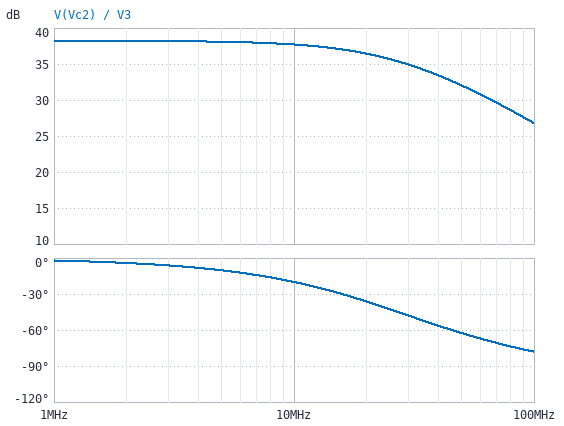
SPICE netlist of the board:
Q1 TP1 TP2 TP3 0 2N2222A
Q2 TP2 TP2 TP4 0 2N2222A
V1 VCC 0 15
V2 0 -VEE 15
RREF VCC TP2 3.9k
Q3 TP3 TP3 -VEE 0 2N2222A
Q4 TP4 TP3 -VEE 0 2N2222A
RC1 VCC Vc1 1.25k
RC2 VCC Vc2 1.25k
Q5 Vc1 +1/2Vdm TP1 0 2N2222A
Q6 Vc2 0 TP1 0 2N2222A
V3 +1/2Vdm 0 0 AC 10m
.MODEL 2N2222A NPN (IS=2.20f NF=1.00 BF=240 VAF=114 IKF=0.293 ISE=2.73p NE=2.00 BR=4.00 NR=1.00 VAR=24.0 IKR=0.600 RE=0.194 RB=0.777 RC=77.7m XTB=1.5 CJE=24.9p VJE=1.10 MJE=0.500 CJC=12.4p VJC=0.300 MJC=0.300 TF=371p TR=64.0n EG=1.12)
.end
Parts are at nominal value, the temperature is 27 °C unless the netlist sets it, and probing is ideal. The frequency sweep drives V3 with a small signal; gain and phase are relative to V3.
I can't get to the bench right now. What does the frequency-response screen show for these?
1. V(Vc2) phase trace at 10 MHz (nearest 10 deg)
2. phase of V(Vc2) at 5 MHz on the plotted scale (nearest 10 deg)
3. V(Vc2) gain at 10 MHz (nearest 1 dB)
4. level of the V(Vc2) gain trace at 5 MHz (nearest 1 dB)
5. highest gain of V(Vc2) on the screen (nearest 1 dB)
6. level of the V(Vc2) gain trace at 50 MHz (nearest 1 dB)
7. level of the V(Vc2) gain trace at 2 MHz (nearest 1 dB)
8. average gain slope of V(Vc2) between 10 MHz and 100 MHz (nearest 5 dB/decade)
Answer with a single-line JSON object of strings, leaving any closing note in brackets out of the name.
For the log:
{"V(Vc2) phase trace at 10 MHz": "-20 deg", "phase of V(Vc2) at 5 MHz on the plotted scale": "-10 deg", "V(Vc2) gain at 10 MHz": "38 dB", "level of the V(Vc2) gain trace at 5 MHz": "38 dB", "highest gain of V(Vc2) on the screen": "38 dB", "level of the V(Vc2) gain trace at 50 MHz": "32 dB", "level of the V(Vc2) gain trace at 2 MHz": "38 dB", "average gain slope of V(Vc2) between 10 MHz and 100 MHz": "-10 dB/decade"}
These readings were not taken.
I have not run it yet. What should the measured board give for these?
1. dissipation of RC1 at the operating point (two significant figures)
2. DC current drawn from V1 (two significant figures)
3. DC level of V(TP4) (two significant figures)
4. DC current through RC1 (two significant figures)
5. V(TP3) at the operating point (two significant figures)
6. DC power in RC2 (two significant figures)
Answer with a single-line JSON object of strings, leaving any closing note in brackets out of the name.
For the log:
{"dissipation of RC1 at the operating point": "17 mW", "DC current drawn from V1": "15 mA", "DC level of V(TP4)": "-14 V", "DC current through RC1": "3.6 mA", "V(TP3) at the operating point": "-14 V", "DC power in RC2": "17 mW"}
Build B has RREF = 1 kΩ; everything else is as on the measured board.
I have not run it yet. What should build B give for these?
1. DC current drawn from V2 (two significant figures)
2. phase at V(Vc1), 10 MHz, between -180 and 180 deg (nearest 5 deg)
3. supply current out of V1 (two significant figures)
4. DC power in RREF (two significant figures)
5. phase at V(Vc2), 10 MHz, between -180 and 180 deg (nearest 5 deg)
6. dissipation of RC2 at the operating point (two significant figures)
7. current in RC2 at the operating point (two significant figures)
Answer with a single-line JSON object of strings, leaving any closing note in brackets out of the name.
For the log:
{"DC current drawn from V2": "57 mA", "phase at V(Vc1), 10 MHz, between -180 and 180 deg": "15 deg", "supply current out of V1": "54 mA", "DC power in RREF": "810 mW", "phase at V(Vc2), 10 MHz, between -180 and 180 deg": "-45 deg", "dissipation of RC2 at the operating point": "200 mW", "current in RC2 at the operating point": "13 mA"}
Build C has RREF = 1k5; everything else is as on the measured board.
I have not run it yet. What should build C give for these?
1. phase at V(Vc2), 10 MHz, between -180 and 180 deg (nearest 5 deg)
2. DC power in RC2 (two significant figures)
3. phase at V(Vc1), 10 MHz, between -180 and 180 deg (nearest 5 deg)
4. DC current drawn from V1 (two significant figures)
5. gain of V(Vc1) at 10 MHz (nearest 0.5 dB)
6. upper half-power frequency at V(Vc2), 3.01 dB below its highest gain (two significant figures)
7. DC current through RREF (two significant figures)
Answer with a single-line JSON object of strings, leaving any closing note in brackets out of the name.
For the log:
{"phase at V(Vc2), 10 MHz, between -180 and 180 deg": "-30 deg", "DC power in RC2": "110 mW", "phase at V(Vc1), 10 MHz, between -180 and 180 deg": "150 deg", "DC current drawn from V1": "38 mA", "gain of V(Vc1) at 10 MHz": "44.5 dB", "upper half-power frequency at V(Vc2), 3.01 dB below its highest gain": "19 MHz", "DC current through RREF": "19 mA"}
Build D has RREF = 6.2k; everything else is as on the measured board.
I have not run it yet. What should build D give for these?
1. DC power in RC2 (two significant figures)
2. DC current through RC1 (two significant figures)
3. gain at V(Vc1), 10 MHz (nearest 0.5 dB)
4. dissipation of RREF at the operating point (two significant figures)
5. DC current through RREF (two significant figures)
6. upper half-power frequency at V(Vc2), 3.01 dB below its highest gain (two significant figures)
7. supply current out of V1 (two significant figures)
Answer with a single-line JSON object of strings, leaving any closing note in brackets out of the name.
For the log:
{"DC power in RC2": "6.6 mW", "DC current through RC1": "2.3 mA", "gain at V(Vc1), 10 MHz": "34.0 dB", "dissipation of RREF at the operating point": "130 mW", "DC current through RREF": "4.6 mA", "upper half-power frequency at V(Vc2), 3.01 dB below its highest gain": "30 MHz", "supply current out of V1": "9.2 mA"}
